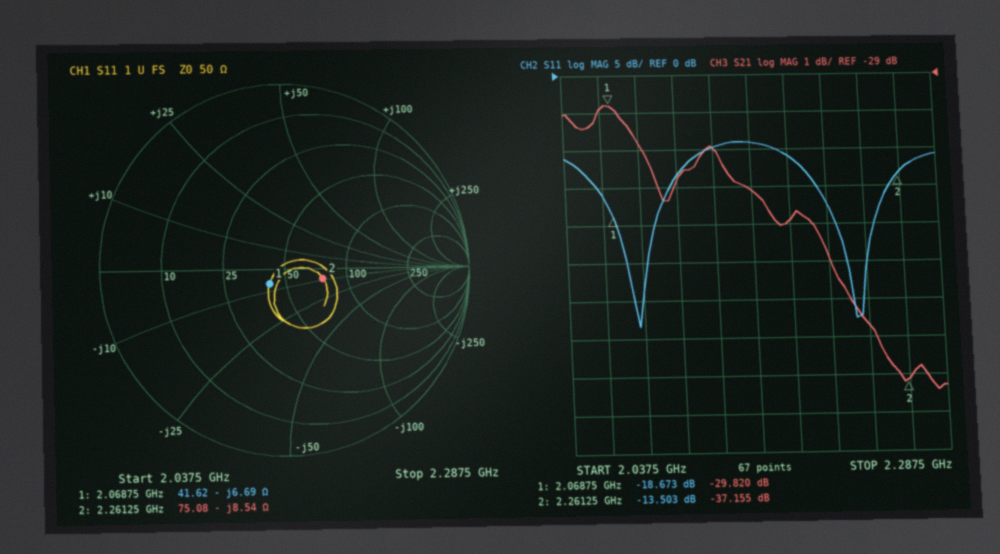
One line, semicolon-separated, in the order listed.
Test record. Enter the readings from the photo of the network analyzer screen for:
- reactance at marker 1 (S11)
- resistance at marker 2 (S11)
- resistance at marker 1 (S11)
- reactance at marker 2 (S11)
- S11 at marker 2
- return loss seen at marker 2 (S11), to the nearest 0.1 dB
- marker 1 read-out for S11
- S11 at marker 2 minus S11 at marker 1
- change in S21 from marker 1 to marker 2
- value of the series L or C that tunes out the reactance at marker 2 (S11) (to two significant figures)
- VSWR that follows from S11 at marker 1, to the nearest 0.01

-6.69 Ω; 75.08 Ω; 41.62 Ω; -8.54 Ω; -13.503 dB; 13.5 dB; -18.673 dB; 5.170 dB; -7.335 dB; 600 pH; 1.26
